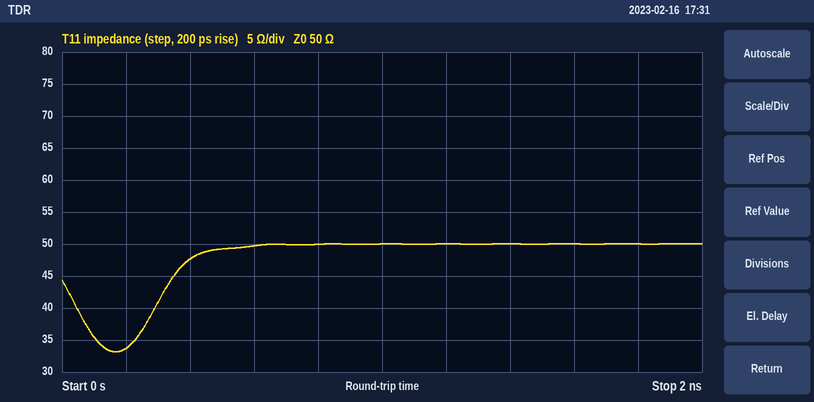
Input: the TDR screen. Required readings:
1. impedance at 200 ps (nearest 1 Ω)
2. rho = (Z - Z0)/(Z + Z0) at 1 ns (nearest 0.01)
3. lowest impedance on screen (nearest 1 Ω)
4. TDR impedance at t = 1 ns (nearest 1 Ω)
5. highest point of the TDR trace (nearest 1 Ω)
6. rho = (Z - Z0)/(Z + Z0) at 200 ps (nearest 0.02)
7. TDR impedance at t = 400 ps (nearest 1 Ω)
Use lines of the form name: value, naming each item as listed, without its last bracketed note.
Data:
impedance at 200 ps: 34 Ω
rho = (Z - Z0)/(Z + Z0) at 1 ns: 0.00
lowest impedance on screen: 33 Ω
TDR impedance at t = 1 ns: 50 Ω
highest point of the TDR trace: 50 Ω
rho = (Z - Z0)/(Z + Z0) at 200 ps: -0.20
TDR impedance at t = 400 ps: 48 Ω
